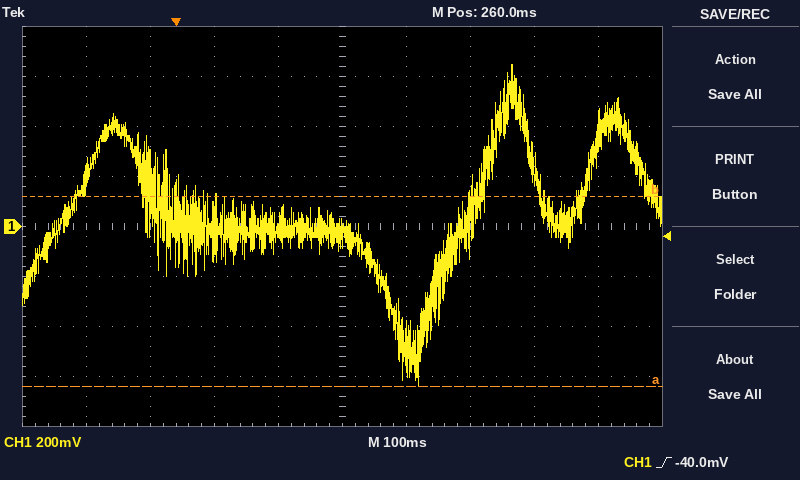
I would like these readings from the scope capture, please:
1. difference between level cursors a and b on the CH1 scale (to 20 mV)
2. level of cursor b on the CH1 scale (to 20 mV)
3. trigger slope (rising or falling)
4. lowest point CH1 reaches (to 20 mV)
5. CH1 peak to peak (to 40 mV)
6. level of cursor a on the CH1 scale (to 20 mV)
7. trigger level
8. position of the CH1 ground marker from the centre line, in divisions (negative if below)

760 mV
120 mV
rising
-640 mV
1.28 V
-640 mV
-40.0 mV
0.0 div
